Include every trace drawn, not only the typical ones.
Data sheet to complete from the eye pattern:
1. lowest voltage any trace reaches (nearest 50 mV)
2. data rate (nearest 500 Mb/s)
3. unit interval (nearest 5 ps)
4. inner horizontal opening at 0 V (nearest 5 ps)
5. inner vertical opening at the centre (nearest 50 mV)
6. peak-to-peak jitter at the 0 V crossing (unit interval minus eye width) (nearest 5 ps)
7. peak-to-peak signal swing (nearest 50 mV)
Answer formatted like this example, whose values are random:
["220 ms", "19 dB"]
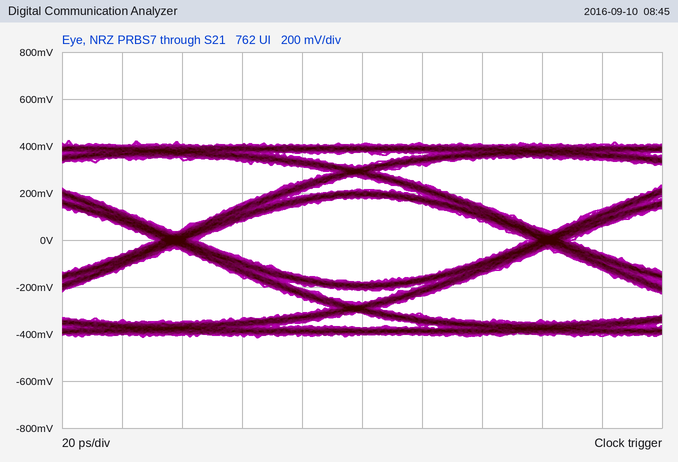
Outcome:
["-400 mV", "8.0 Gb/s", "125 ps", "110 ps", "350 mV", "15 ps", "850 mV"]
